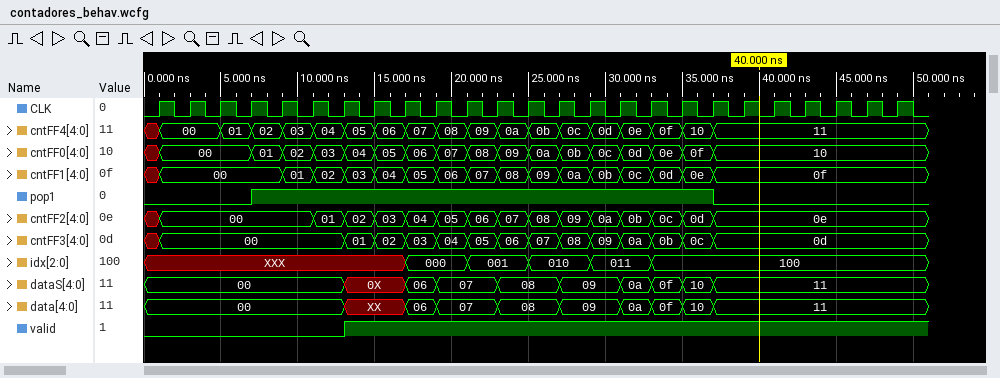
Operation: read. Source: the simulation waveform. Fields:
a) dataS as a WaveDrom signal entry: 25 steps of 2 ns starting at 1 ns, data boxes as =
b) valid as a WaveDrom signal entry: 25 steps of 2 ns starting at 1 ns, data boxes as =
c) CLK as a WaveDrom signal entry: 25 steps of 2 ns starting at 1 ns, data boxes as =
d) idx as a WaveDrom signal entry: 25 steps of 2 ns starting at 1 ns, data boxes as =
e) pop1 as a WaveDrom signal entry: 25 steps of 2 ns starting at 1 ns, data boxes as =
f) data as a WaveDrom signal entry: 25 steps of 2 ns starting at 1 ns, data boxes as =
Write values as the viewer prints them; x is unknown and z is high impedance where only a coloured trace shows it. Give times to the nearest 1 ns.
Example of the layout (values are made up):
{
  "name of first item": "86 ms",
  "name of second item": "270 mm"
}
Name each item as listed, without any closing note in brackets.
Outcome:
{
  "dataS as a WaveDrom signal entry: 25 steps of 2 ns starting at 1 ns, data boxes as =": "{name: 'dataS', wave: '=.....=.==.=.=.====......', data: '00 0X 06 07 08 09 0a 0f 10 11'}",
  "valid as a WaveDrom signal entry: 25 steps of 2 ns starting at 1 ns, data boxes as =": "{name: 'valid', wave: '0.....1..................'}",
  "CLK as a WaveDrom signal entry: 25 steps of 2 ns starting at 1 ns, data boxes as =": "{name: 'CLK', wave: 'p........................'}",
  "idx as a WaveDrom signal entry: 25 steps of 2 ns starting at 1 ns, data boxes as =": "{name: 'idx', wave: 'x.......=.=.=.=.=........', data: '000 001 010 011 100'}",
  "pop1 as a WaveDrom signal entry: 25 steps of 2 ns starting at 1 ns, data boxes as =": "{name: 'pop1', wave: '0..1..............0......'}",
  "data as a WaveDrom signal entry: 25 steps of 2 ns starting at 1 ns, data boxes as =": "{name: 'data', wave: '=.....x.==.=.=.====......', data: '00 06 07 08 09 0a 0f 10 11'}"
}
